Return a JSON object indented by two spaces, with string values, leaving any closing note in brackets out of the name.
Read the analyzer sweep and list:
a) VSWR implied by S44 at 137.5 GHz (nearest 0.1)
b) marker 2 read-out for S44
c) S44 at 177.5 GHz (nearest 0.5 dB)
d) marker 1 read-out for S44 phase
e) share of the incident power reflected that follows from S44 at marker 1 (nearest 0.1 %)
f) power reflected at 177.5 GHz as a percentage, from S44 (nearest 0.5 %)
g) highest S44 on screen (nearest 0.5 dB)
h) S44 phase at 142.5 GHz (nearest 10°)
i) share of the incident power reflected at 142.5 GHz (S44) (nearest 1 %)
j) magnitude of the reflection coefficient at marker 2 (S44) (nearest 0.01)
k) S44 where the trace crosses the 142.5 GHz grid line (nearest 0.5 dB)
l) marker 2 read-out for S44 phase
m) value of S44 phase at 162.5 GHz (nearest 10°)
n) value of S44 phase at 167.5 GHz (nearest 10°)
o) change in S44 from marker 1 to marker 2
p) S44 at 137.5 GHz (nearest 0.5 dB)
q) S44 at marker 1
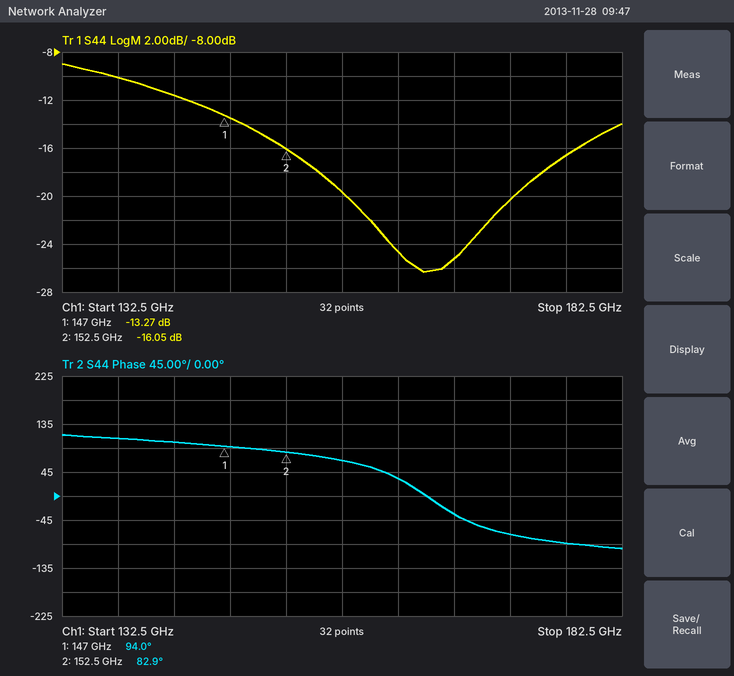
{
  "VSWR implied by S44 at 137.5 GHz": "1.9",
  "marker 2 read-out for S44": "-16.05 dB",
  "S44 at 177.5 GHz": "-16.5 dB",
  "marker 1 read-out for S44 phase": "94.0°",
  "share of the incident power reflected that follows from S44 at marker 1": "4.7 %",
  "power reflected at 177.5 GHz as a percentage, from S44": "2.0 %",
  "highest S44 on screen": "-9.0 dB",
  "S44 phase at 142.5 GHz": "100°",
  "share of the incident power reflected at 142.5 GHz (S44)": "7 %",
  "magnitude of the reflection coefficient at marker 2 (S44)": "0.16",
  "S44 where the trace crosses the 142.5 GHz grid line": "-11.5 dB",
  "marker 2 read-out for S44 phase": "82.9°",
  "value of S44 phase at 162.5 GHz": "30°",
  "value of S44 phase at 167.5 GHz": "-30°",
  "change in S44 from marker 1 to marker 2": "-2.78 dB",
  "S44 at 137.5 GHz": "-10.0 dB",
  "S44 at marker 1": "-13.27 dB"
}
